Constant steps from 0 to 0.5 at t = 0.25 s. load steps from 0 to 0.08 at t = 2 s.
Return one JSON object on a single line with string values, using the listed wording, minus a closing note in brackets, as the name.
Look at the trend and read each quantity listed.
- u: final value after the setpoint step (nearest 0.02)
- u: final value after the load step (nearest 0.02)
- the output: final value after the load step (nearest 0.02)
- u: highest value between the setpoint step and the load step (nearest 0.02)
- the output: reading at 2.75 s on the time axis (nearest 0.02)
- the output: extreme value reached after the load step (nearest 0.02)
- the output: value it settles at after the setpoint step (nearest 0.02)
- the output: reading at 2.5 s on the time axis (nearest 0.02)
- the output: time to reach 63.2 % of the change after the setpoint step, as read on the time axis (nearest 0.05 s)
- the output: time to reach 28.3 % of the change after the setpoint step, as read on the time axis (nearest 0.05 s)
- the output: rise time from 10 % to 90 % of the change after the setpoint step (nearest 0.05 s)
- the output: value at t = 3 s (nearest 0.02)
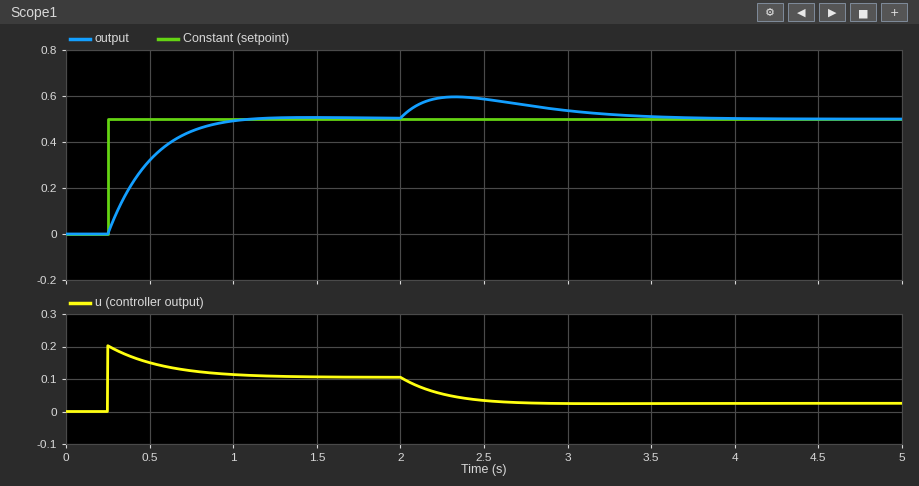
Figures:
{"u: final value after the setpoint step": "0.10", "u: final value after the load step": "0.02", "the output: final value after the load step": "0.50", "u: highest value between the setpoint step and the load step": "0.20", "the output: reading at 2.75 s on the time axis": "0.56", "the output: extreme value reached after the load step": "0.60", "the output: value it settles at after the setpoint step": "0.50", "the output: reading at 2.5 s on the time axis": "0.58", "the output: time to reach 63.2 % of the change after the setpoint step, as read on the time axis": "0.50 s", "the output: time to reach 28.3 % of the change after the setpoint step, as read on the time axis": "0.35 s", "the output: rise time from 10 % to 90 % of the change after the setpoint step": "0.50 s", "the output: value at t = 3 s": "0.54"}
